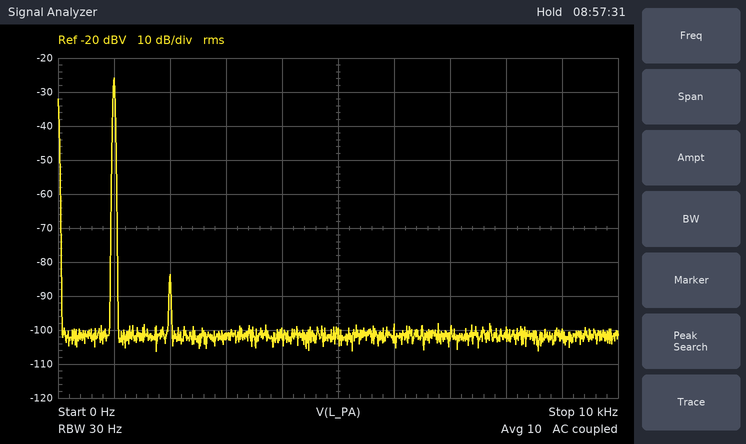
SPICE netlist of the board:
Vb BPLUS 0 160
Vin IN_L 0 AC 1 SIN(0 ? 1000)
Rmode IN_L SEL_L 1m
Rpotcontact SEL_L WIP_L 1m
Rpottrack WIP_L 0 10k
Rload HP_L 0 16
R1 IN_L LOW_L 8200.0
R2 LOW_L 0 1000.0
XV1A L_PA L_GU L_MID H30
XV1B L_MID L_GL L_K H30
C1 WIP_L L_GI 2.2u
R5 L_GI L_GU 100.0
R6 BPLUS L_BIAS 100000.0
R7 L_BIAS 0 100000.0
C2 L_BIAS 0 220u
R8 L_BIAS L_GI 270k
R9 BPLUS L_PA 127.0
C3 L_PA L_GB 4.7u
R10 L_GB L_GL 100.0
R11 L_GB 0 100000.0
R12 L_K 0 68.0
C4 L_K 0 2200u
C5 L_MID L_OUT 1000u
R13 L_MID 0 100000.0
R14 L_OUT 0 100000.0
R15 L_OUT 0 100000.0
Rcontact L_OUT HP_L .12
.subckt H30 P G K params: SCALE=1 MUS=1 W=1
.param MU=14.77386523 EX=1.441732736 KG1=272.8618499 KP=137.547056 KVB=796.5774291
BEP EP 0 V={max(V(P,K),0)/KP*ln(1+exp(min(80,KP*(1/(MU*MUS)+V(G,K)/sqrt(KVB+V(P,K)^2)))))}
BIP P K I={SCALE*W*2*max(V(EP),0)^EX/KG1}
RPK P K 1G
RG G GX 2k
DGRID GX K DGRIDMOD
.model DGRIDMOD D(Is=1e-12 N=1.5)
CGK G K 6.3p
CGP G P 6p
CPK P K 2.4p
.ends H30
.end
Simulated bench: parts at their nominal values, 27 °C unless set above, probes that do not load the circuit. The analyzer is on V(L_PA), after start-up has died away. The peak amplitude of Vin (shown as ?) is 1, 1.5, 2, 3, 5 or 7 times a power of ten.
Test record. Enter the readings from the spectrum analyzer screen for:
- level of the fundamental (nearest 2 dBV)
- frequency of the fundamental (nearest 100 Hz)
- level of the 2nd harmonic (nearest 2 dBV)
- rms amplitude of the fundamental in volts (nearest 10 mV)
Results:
-26 dBV
1.0 kHz
-84 dBV
50 mV
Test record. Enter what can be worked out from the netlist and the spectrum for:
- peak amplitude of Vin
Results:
70 mV
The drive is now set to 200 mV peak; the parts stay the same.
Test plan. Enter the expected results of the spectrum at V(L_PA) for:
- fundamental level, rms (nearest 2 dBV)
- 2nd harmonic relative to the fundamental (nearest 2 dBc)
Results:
-16 dBV
-48 dBc
